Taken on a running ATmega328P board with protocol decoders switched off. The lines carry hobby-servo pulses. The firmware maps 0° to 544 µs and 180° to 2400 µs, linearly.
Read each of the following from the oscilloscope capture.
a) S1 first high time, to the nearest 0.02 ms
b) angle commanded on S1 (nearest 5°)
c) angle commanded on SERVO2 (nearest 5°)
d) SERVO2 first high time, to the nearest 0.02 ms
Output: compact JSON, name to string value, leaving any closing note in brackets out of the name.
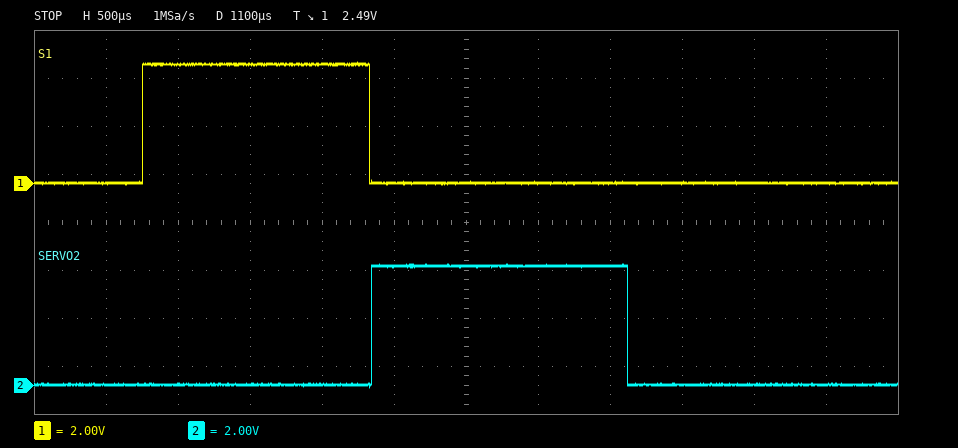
{"S1 first high time, to the nearest 0.02 ms": "1.58 ms", "angle commanded on S1": "100°", "angle commanded on SERVO2": "120°", "SERVO2 first high time, to the nearest 0.02 ms": "1.78 ms"}
